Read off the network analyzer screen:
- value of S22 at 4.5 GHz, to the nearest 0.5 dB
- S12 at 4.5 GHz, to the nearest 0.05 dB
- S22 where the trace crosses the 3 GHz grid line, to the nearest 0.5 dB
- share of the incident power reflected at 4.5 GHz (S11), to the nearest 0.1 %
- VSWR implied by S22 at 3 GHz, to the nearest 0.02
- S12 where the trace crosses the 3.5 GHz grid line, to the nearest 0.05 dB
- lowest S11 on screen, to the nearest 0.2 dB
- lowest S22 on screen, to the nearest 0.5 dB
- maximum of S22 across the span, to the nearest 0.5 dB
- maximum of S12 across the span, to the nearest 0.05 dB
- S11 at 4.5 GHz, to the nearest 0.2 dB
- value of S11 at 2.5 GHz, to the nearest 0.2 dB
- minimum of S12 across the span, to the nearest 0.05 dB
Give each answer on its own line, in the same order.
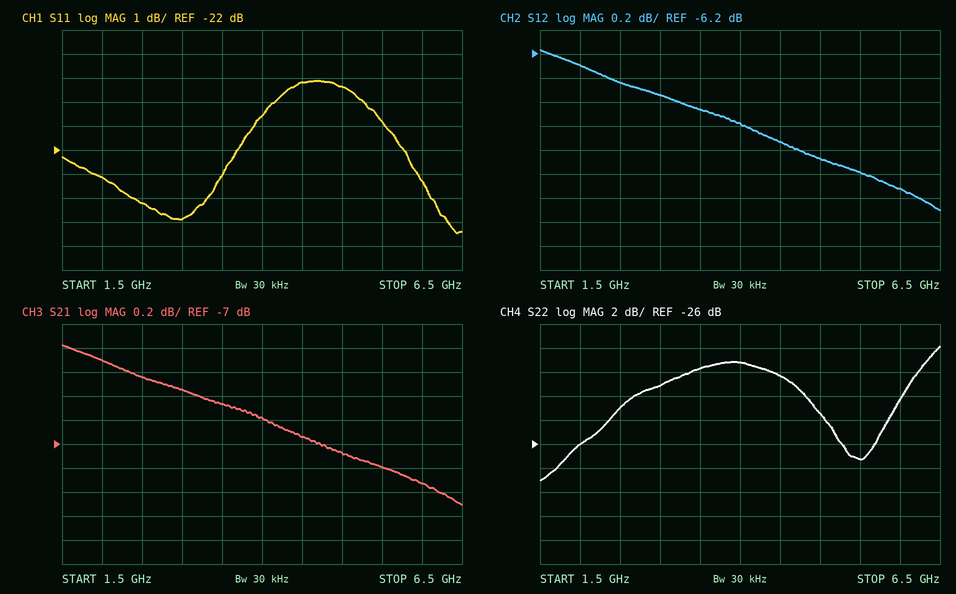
-20.5 dB
-6.95 dB
-21.0 dB
1.2 %
1.20
-6.65 dB
-25.4 dB
-29.0 dB
-18.0 dB
-6.15 dB
-19.2 dB
-24.2 dB
-7.50 dB
